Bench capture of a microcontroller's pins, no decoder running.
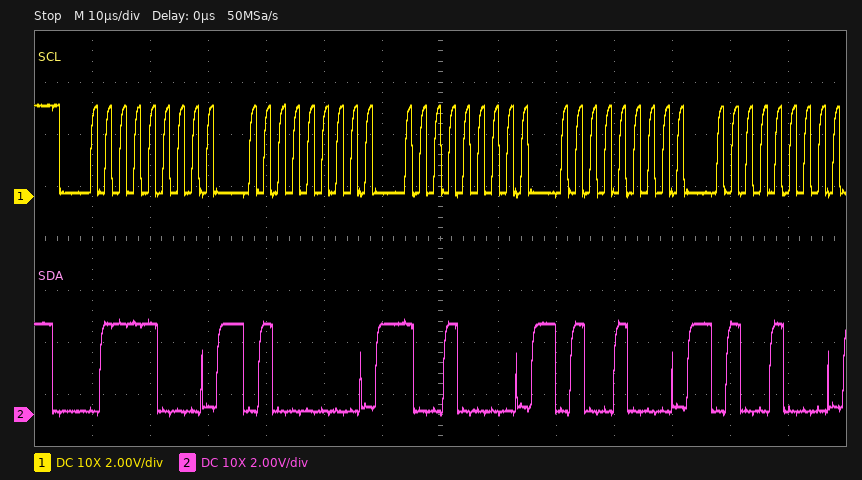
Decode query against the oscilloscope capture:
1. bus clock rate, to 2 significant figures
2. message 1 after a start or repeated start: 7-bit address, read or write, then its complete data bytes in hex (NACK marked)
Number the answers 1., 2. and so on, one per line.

1. 400 kHz
2. 0x3C write: 40 90 48 48
